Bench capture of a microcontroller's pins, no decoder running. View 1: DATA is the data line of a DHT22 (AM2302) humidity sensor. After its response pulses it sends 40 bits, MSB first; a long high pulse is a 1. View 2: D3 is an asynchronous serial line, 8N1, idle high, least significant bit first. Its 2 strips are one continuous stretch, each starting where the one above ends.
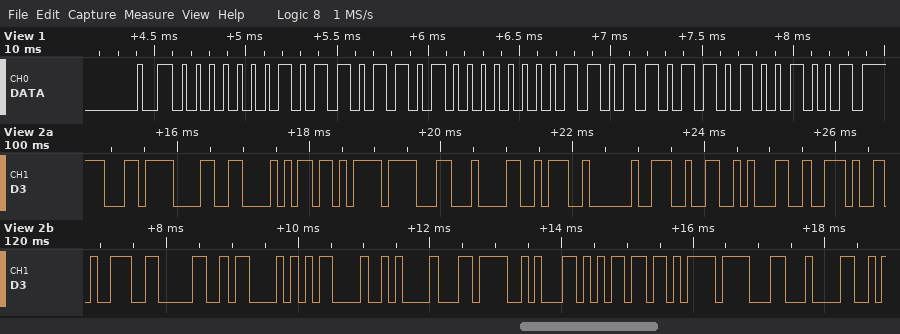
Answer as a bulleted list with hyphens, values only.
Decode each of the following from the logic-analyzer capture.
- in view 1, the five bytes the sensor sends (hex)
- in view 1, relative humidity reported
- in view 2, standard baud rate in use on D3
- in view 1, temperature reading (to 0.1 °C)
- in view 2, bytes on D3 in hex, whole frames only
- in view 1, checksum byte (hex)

- 01 6D 00 DB 49
- 36.5 %
- 9600 baud
- 21.9 °C
- EC 98 A8 EB 8F 84 3A 20 32 31 2E 39 30 43 0D 0A EC 8A B5 EB 8F 84
- 0x49
